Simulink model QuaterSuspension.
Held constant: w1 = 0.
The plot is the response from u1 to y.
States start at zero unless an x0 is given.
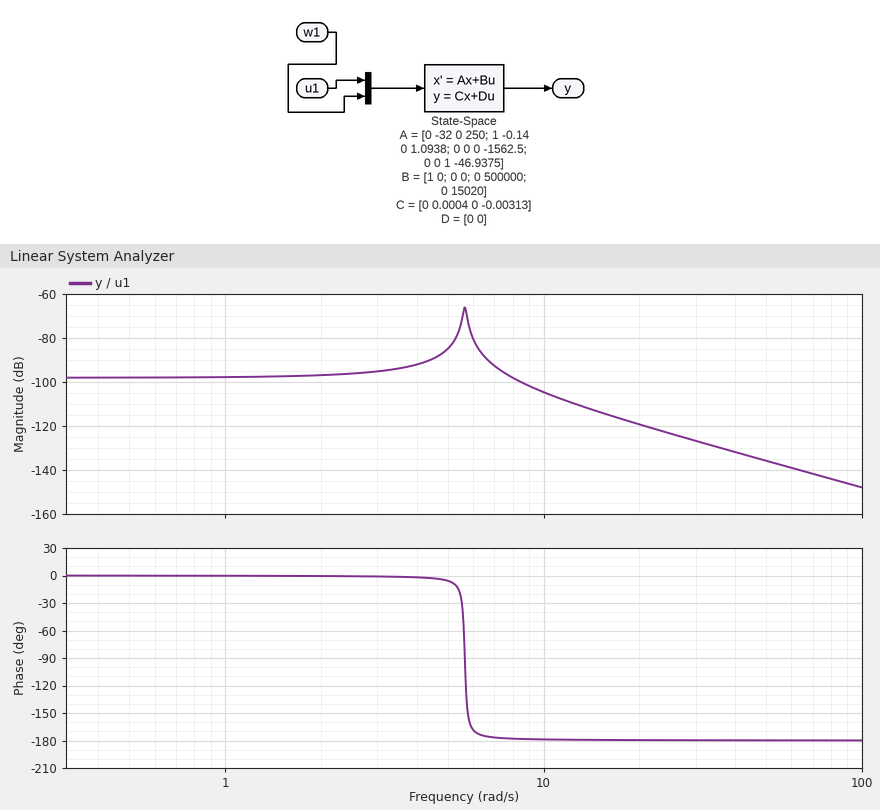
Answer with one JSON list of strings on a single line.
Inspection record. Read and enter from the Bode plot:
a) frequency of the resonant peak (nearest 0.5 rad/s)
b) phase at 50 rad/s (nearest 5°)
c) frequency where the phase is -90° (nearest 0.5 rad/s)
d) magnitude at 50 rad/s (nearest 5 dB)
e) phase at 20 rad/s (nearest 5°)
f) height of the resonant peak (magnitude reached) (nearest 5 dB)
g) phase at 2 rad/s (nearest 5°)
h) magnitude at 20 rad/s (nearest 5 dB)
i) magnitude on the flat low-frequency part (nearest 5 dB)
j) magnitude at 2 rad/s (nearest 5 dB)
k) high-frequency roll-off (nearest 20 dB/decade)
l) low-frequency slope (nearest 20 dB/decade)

["5.5 rad/s", "-180°", "5.5 rad/s", "-135 dB", "-180°", "-65 dB", "0°", "-120 dB", "-100 dB", "-95 dB", "-40 dB/decade", "0 dB/decade"]
